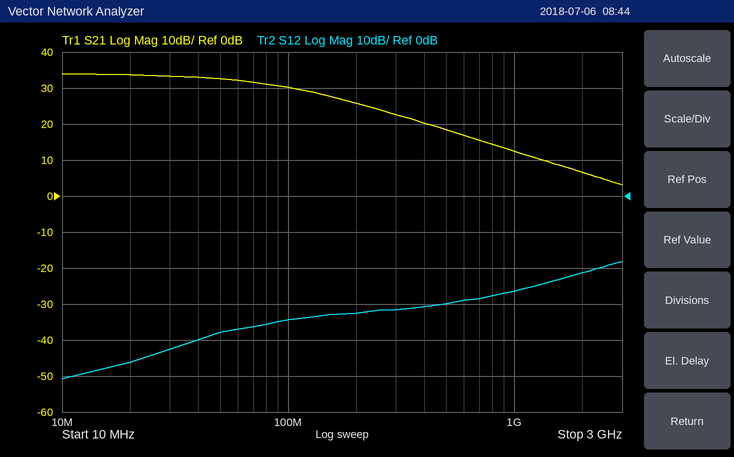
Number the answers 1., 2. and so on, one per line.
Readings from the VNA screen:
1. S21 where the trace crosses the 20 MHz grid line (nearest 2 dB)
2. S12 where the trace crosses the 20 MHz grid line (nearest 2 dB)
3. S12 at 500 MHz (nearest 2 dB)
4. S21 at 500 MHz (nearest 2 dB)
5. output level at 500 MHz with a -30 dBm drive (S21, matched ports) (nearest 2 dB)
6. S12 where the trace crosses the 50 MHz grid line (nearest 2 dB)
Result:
1. 34 dB
2. -46 dB
3. -30 dB
4. 18 dB
5. -12 dBm
6. -38 dB
